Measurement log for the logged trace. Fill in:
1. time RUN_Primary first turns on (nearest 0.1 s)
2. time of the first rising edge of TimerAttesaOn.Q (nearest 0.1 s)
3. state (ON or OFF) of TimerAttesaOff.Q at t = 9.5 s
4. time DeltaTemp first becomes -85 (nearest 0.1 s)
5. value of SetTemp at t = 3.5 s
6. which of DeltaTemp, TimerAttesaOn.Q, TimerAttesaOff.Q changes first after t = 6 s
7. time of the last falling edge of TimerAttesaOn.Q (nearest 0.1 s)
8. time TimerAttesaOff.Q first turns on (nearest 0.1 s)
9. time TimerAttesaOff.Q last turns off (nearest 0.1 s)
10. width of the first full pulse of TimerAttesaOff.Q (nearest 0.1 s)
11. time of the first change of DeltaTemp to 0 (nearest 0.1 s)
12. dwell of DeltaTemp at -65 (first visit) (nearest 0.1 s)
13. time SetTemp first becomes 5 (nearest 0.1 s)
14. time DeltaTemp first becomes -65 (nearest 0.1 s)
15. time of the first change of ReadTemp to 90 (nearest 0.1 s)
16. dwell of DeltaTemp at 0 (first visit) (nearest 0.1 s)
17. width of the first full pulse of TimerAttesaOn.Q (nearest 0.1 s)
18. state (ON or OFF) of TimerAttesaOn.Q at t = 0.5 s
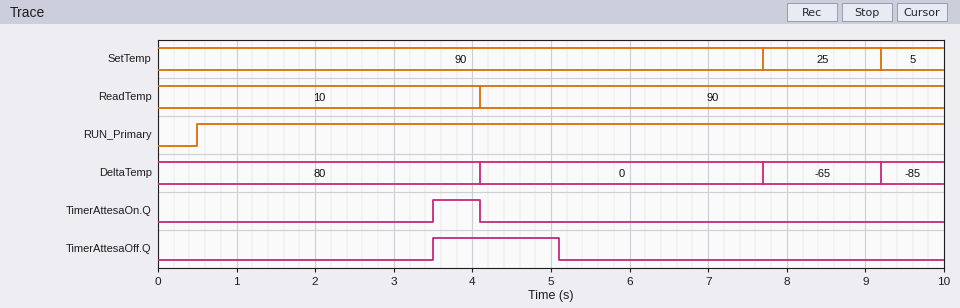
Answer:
0.5 s
3.5 s
OFF
9.2 s
90
DeltaTemp
4.1 s
3.5 s
5.1 s
1.6 s
4.1 s
1.5 s
9.2 s
7.7 s
4.1 s
3.6 s
0.6 s
OFF
